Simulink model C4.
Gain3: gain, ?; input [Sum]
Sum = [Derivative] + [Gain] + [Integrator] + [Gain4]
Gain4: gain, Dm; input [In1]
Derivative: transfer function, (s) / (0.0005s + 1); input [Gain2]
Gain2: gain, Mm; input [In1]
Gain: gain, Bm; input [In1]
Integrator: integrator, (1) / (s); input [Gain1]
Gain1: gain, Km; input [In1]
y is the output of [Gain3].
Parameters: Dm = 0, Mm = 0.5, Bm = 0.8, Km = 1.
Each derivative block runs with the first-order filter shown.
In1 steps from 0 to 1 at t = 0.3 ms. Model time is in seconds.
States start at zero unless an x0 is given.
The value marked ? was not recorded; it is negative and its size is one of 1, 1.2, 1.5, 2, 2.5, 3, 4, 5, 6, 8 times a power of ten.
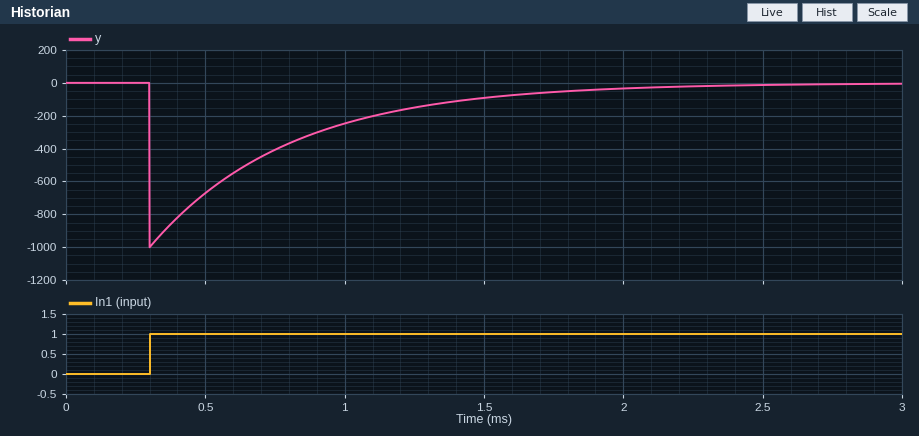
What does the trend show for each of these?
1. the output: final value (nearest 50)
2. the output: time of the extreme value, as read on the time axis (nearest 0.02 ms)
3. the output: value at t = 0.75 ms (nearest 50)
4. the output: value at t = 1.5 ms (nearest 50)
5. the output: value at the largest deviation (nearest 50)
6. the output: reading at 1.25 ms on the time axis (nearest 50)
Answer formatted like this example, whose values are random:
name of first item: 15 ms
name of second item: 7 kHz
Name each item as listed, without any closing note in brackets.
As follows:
the output: final value: 0
the output: time of the extreme value, as read on the time axis: 0.30 ms
the output: value at t = 0.75 ms: -400
the output: value at t = 1.5 ms: -100
the output: value at the largest deviation: -1000
the output: reading at 1.25 ms on the time axis: -150
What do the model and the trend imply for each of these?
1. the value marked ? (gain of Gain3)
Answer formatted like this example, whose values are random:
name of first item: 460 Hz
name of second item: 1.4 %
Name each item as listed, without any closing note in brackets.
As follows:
the value marked ?: -1
